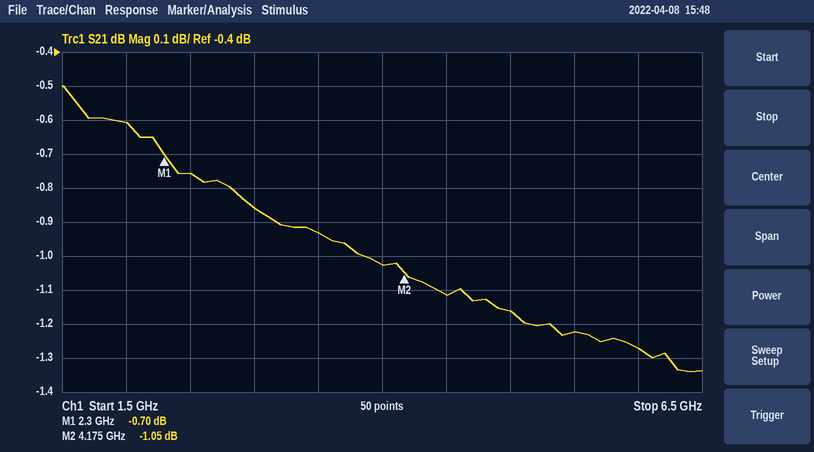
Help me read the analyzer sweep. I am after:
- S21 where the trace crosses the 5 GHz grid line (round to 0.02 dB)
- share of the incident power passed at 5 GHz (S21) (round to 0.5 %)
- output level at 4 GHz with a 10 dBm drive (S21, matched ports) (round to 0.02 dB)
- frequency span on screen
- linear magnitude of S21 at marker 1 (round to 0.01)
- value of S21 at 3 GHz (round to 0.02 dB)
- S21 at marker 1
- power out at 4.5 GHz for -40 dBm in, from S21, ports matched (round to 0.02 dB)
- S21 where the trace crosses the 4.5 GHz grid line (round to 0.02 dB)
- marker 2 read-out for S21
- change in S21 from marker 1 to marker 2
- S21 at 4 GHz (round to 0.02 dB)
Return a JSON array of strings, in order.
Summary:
["-1.16 dB", "76.5 %", "8.98 dBm", "5 GHz", "0.92", "-0.86 dB", "-0.70 dB", "-41.12 dBm", "-1.12 dB", "-1.05 dB", "-0.35 dB", "-1.02 dB"]
